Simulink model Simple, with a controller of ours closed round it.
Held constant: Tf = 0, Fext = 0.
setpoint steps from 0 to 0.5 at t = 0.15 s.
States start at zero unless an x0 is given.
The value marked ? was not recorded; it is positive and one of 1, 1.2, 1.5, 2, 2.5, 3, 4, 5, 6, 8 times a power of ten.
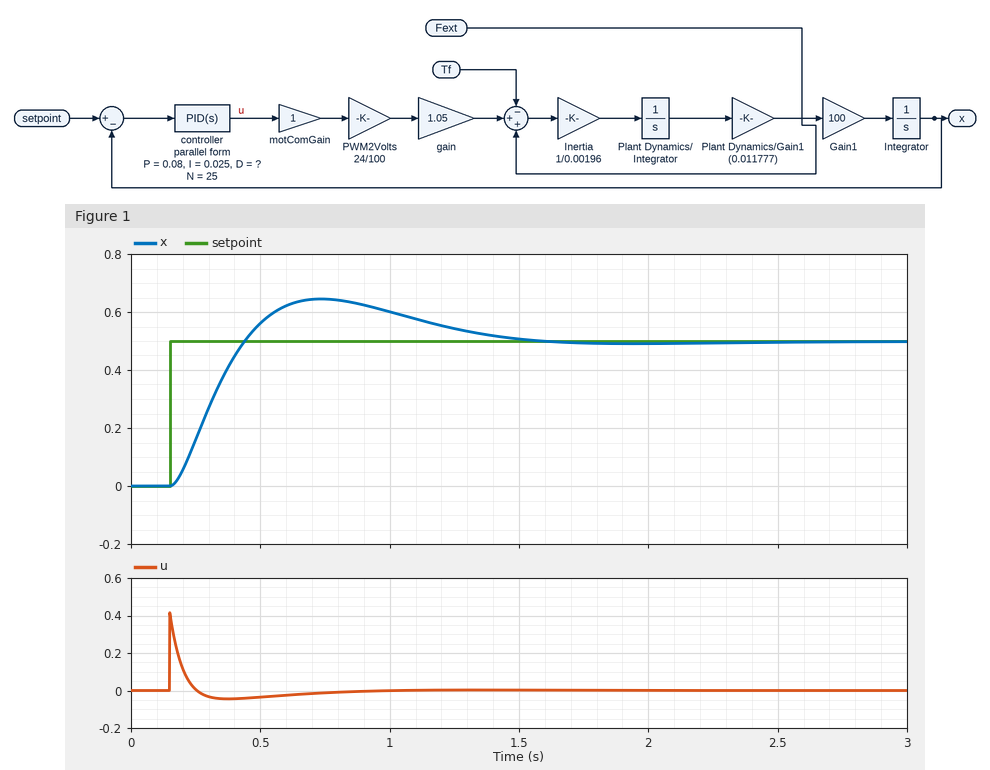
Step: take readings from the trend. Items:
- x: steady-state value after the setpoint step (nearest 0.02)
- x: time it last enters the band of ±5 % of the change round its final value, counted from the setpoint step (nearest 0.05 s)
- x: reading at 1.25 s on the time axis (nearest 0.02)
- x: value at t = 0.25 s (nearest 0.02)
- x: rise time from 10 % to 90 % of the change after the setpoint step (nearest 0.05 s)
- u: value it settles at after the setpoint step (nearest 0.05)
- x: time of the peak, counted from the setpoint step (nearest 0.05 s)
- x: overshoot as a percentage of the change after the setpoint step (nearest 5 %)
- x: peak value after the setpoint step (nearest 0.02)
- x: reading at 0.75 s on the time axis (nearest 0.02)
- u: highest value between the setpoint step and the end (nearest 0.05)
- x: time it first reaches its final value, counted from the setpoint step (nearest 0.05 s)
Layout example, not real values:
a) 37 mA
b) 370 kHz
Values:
a) 0.50
b) 1.20 s
c) 0.54
d) 0.16
e) 0.20 s
f) 0.00
g) 0.60 s
h) 30 %
i) 0.64
j) 0.64
k) 0.40
l) 0.30 s
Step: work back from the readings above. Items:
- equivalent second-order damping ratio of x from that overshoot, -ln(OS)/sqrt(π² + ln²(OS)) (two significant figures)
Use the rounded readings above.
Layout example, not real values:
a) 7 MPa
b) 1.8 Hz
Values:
a) 0.36
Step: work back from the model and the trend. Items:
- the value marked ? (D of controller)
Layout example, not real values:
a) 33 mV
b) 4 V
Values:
a) 0.03
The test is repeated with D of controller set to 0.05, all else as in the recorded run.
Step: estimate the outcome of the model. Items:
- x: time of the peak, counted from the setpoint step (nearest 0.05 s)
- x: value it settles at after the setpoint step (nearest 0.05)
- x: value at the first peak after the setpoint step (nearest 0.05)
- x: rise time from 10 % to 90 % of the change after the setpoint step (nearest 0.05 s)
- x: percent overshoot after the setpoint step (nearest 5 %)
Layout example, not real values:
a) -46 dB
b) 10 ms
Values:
a) 0.40 s
b) 0.50
c) 0.60
d) 0.15 s
e) 15 %
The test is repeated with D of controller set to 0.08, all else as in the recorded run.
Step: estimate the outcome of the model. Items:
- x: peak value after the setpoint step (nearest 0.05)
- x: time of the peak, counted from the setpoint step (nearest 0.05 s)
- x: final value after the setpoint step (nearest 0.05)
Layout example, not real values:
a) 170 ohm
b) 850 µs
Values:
a) 0.55
b) 0.25 s
c) 0.50
